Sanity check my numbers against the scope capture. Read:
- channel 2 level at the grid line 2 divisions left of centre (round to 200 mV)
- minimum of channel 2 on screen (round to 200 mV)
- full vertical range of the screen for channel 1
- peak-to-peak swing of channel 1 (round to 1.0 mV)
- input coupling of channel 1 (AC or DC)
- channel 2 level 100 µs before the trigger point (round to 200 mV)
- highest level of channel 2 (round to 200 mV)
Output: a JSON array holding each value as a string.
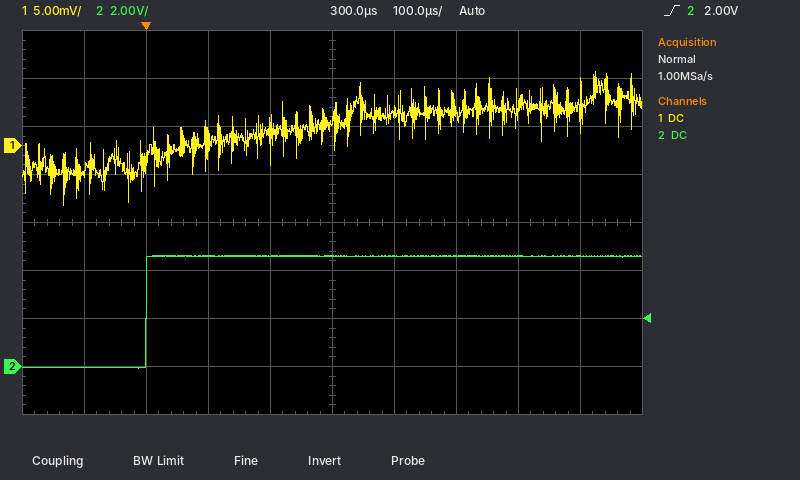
["4.6 V", "0.0 V", "40 mV", "14.0 mV", "DC", "0.0 V", "4.6 V"]
